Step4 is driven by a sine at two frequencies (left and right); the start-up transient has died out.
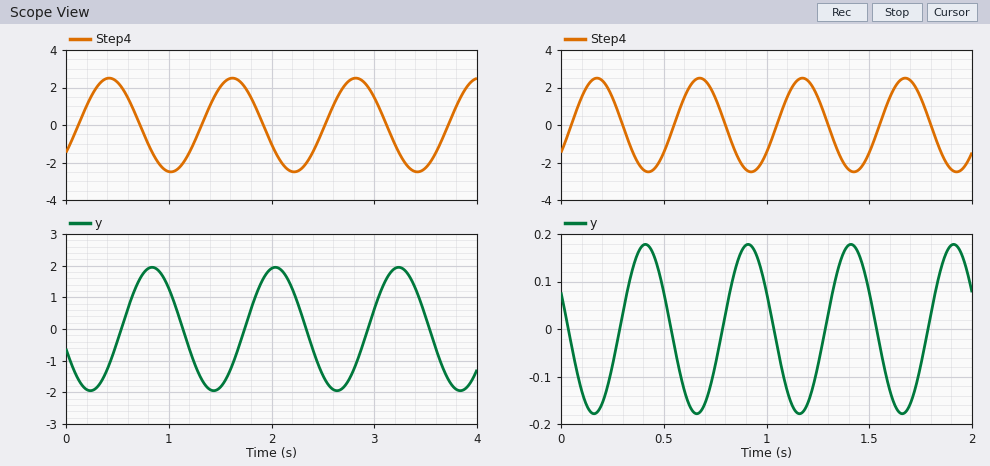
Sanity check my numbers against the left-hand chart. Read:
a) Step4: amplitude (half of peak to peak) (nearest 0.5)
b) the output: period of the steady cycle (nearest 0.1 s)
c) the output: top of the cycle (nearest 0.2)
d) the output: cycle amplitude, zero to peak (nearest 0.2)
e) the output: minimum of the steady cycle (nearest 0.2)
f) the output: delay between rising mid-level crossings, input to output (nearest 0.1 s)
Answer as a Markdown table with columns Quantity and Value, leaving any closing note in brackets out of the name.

| Quantity | Value |
|---|---|
| Step4: amplitude (half of peak to peak) | 2.5 |
| the output: period of the steady cycle | 1.2 s |
| the output: top of the cycle | 2.0 |
| the output: cycle amplitude, zero to peak | 2.0 |
| the output: minimum of the steady cycle | -2.0 |
| the output: delay between rising mid-level crossings, input to output | 0.4 s |
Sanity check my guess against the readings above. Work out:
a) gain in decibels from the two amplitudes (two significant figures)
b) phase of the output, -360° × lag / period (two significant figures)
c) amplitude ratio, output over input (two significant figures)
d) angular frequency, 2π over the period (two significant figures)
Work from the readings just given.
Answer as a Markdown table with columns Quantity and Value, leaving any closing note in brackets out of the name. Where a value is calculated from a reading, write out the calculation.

| Quantity | Value |
|---|---|
| gain in decibels from the two amplitudes | 20 log10(2 / 2.5) = -1.9 dB |
| phase of the output, -360° × lag / period | -360 × 0.4 / 1.2 = -120° |
| amplitude ratio, output over input | 2 / 2.5 = 0.80 |
| angular frequency, 2π over the period | 2π / 1.2 = 5.2 rad/s |
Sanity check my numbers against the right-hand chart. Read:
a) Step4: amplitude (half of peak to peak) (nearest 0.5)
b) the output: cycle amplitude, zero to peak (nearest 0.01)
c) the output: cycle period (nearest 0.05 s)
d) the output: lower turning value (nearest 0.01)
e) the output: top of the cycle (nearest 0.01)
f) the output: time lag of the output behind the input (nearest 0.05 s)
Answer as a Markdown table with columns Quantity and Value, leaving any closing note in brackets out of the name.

| Quantity | Value |
|---|---|
| Step4: amplitude (half of peak to peak) | 2.5 |
| the output: cycle amplitude, zero to peak | 0.18 |
| the output: cycle period | 0.50 s |
| the output: lower turning value | -0.18 |
| the output: top of the cycle | 0.18 |
| the output: time lag of the output behind the input | 0.25 s |
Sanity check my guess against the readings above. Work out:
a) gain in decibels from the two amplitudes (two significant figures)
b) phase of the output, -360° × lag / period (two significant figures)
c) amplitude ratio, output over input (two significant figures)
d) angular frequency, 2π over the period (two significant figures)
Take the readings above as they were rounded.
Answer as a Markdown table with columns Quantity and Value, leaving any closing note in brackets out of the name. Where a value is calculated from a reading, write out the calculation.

| Quantity | Value |
|---|---|
| gain in decibels from the two amplitudes | 20 log10(0.18 / 2.5) = -23 dB |
| phase of the output, -360° × lag / period | -360 × 0.25 / 0.5 = -180° |
| amplitude ratio, output over input | 0.18 / 2.5 = 0.072 |
| angular frequency, 2π over the period | 2π / 0.5 = 13 rad/s |
